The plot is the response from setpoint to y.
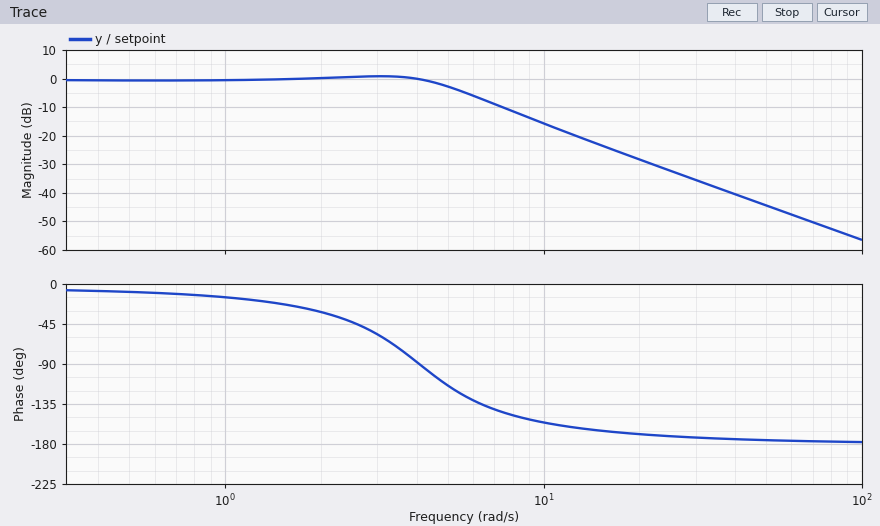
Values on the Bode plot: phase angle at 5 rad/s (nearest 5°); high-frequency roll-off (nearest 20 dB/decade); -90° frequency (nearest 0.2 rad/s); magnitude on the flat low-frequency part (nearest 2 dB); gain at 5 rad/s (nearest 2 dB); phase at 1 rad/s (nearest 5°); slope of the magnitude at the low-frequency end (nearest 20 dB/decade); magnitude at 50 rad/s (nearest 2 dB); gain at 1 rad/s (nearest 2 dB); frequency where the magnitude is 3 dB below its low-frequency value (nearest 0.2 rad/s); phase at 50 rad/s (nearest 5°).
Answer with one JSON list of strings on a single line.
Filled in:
["-115°", "-40 dB/decade", "4.0 rad/s", "0 dB", "-2 dB", "-15°", "0 dB/decade", "-44 dB", "0 dB", "5.2 rad/s", "-175°"]
